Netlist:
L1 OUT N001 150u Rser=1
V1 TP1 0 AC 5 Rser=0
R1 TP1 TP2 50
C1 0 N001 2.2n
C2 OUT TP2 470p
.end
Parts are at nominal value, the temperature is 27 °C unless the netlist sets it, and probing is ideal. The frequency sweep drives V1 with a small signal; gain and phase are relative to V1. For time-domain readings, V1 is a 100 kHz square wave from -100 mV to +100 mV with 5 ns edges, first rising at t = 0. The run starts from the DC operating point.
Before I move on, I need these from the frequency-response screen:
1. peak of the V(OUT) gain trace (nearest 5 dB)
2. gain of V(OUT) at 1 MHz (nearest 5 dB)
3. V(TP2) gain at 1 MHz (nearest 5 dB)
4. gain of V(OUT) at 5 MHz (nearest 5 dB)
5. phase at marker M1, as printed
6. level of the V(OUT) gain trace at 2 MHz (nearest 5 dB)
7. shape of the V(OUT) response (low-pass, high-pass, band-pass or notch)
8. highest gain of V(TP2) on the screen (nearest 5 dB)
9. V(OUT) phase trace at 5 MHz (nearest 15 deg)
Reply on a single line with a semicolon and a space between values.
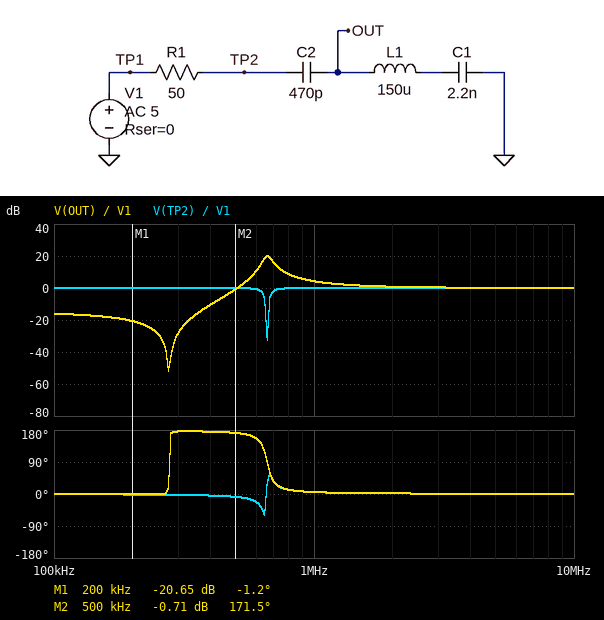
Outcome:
20 dB; 5 dB; 0 dB; 0 dB; -1.2 deg; 0 dB; band-pass; 0 dB; 0 deg
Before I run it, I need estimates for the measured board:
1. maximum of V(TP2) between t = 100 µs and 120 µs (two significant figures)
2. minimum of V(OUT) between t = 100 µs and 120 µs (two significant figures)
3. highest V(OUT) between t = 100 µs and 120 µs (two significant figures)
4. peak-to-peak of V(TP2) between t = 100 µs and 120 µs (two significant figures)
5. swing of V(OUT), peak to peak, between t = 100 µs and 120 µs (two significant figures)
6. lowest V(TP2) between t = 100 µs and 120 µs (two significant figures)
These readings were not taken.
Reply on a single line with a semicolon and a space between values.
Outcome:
110 mV; -170 mV; 200 mV; 230 mV; 370 mV; -110 mV
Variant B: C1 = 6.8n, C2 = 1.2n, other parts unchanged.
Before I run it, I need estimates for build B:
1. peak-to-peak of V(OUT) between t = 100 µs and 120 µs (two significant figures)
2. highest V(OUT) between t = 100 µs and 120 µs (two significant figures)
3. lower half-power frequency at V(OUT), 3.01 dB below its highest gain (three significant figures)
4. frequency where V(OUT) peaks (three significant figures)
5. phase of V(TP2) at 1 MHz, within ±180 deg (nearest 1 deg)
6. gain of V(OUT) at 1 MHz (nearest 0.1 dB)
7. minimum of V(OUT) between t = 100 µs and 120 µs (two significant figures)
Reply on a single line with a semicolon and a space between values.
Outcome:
270 mV; 150 mV; 385 kHz; 409 kHz; 4 deg; 1.3 dB; -120 mV
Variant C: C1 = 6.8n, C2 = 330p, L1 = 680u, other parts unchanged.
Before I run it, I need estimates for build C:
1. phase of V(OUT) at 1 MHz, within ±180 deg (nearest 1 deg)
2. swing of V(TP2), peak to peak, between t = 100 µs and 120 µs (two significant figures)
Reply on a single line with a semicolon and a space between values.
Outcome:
1 deg; 210 mV
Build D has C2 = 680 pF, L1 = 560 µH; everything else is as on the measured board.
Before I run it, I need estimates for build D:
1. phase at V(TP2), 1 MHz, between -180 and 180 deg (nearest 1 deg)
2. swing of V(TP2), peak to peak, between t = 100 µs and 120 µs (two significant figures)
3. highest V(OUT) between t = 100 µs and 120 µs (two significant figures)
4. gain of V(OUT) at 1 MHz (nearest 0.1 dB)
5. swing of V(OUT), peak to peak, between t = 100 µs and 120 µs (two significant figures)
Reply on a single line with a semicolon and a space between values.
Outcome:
1 deg; 270 mV; 660 mV; 0.6 dB; 1.3 V
